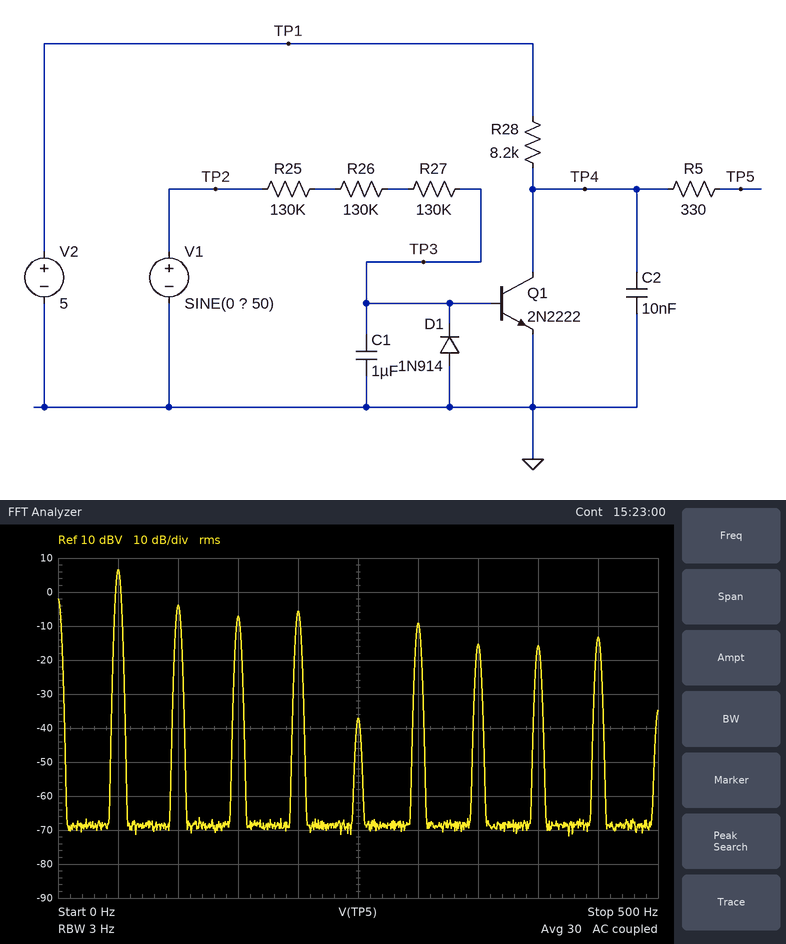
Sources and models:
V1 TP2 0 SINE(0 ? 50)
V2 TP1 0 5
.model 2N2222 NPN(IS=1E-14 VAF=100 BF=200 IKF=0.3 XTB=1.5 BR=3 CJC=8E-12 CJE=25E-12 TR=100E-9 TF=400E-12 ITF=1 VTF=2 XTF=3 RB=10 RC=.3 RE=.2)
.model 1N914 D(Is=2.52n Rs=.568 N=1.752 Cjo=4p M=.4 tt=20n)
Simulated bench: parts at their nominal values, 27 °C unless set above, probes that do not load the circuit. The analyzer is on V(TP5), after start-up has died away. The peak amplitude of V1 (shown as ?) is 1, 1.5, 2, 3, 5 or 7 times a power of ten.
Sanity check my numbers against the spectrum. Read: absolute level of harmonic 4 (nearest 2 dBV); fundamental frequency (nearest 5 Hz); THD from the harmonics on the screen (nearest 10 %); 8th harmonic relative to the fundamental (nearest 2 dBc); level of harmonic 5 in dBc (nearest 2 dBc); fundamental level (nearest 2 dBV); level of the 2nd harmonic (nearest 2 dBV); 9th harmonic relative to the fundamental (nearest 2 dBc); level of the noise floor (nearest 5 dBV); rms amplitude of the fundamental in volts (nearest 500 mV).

-6 dBV
50 Hz
50 %
-22 dBc
-44 dBc
6 dBV
-4 dBV
-20 dBc
-70 dBV
2.0 V
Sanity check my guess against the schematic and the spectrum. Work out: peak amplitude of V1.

500 V
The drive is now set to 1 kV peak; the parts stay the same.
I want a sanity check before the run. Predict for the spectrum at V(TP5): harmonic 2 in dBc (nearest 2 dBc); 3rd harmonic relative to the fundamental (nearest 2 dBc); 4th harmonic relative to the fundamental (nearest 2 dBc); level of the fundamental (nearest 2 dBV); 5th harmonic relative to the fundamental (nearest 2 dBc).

-14 dBc
-12 dBc
-14 dBc
6 dBV
-20 dBc
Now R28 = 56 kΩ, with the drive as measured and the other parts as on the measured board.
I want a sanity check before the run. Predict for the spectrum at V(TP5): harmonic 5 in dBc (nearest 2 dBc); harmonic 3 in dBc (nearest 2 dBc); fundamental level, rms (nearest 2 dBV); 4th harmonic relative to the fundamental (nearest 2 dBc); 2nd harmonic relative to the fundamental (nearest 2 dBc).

-22 dBc
-12 dBc
6 dBV
-14 dBc
-14 dBc
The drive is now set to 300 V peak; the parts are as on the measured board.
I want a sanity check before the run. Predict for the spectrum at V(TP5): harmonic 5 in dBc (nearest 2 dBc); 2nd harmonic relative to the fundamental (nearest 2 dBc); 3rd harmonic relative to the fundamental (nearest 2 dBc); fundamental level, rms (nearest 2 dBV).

-20 dBc
-8 dBc
-18 dBc
6 dBV
